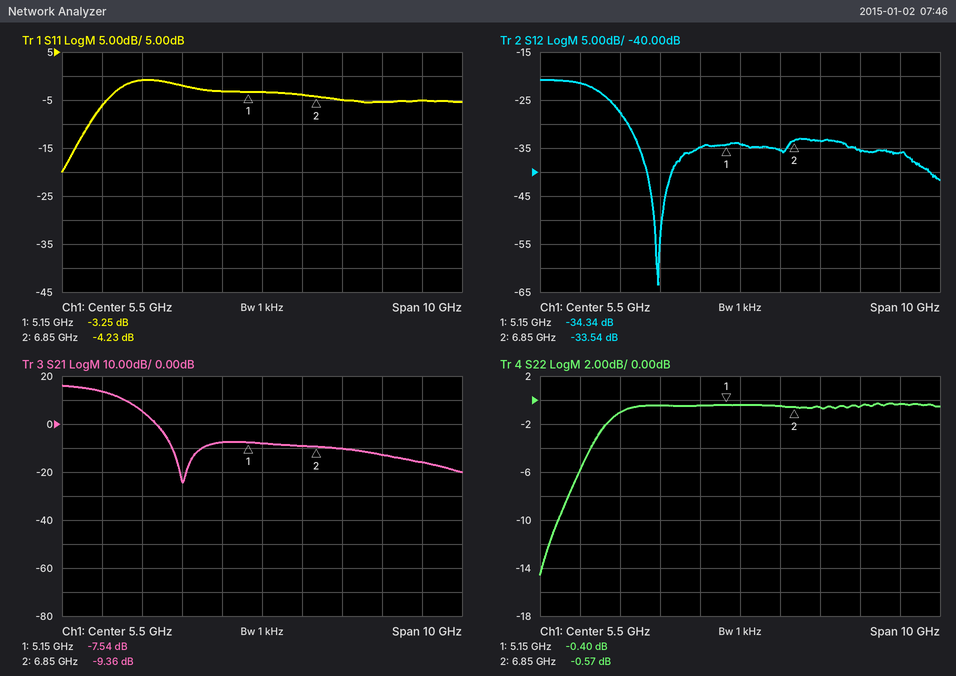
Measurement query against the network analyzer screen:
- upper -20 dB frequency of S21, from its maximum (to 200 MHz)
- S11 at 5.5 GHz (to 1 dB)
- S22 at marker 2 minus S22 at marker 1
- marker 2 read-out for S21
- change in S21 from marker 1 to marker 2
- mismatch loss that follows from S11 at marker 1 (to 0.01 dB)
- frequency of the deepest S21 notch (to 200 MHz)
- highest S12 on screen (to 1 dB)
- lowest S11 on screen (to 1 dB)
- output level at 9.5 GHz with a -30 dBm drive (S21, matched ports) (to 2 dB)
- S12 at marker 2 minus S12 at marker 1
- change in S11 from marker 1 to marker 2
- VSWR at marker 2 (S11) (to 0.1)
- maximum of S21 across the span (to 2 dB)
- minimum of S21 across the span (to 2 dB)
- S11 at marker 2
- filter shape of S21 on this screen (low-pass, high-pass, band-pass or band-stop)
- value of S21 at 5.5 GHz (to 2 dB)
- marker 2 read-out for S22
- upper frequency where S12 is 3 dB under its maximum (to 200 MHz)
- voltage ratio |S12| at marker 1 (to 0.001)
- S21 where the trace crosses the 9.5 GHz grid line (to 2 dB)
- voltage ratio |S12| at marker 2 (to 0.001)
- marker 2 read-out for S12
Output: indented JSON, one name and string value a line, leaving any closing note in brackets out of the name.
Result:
{
  "upper -20 dB frequency of S21, from its maximum": "3.0 GHz",
  "S11 at 5.5 GHz": "-3 dB",
  "S22 at marker 2 minus S22 at marker 1": "-0.17 dB",
  "marker 2 read-out for S21": "-9.36 dB",
  "change in S21 from marker 1 to marker 2": "-1.82 dB",
  "mismatch loss that follows from S11 at marker 1": "2.78 dB",
  "frequency of the deepest S21 notch": "3.6 GHz",
  "highest S12 on screen": "-21 dB",
  "lowest S11 on screen": "-20 dB",
  "output level at 9.5 GHz with a -30 dBm drive (S21, matched ports)": "-46 dBm",
  "S12 at marker 2 minus S12 at marker 1": "0.80 dB",
  "change in S11 from marker 1 to marker 2": "-0.98 dB",
  "VSWR at marker 2 (S11)": "4.2",
  "maximum of S21 across the span": "16 dB",
  "minimum of S21 across the span": "-24 dB",
  "S11 at marker 2": "-4.23 dB",
  "filter shape of S21 on this screen": "low-pass",
  "value of S21 at 5.5 GHz": "-8 dB",
  "marker 2 read-out for S22": "-0.57 dB",
  "upper frequency where S12 is 3 dB under its maximum": "2.0 GHz",
  "voltage ratio |S12| at marker 1": "0.019",
  "S21 where the trace crosses the 9.5 GHz grid line": "-16 dB",
  "voltage ratio |S12| at marker 2": "0.021",
  "marker 2 read-out for S12": "-33.54 dB"
}
